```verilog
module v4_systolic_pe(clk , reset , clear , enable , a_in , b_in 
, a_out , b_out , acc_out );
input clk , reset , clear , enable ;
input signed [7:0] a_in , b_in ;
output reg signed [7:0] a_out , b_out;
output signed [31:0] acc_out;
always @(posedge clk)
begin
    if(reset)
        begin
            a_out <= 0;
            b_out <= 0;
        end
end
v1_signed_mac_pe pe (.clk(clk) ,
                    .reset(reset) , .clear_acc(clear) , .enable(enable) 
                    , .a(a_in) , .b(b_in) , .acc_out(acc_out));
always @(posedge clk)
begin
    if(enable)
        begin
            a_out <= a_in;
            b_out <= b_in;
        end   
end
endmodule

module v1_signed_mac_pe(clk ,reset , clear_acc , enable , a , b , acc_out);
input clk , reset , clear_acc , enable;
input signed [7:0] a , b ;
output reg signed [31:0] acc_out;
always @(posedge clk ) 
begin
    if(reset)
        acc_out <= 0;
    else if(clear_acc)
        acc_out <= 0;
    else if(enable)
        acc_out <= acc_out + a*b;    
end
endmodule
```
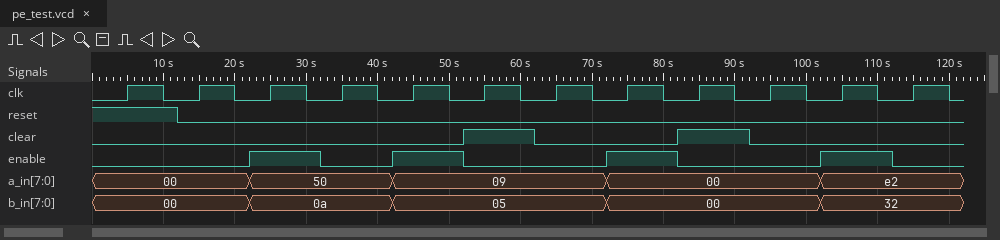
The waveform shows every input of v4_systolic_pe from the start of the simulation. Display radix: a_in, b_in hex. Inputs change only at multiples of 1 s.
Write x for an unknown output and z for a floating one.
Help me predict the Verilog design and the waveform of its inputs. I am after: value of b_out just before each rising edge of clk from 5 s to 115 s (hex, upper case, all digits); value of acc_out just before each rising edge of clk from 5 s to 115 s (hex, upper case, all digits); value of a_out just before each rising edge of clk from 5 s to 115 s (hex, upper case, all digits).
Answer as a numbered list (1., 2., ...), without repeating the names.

1. x, 00, 00, 0A, 0A, 05, 05, 05, 00, 00, 00, 32
2. x, 00000000, 00000000, 00000320, 00000320, 0000034D, 00000000, 00000000, 00000000, 00000000, 00000000, FFFFFA24
3. x, 00, 00, 50, 50, 09, 09, 09, 00, 00, 00, E2
